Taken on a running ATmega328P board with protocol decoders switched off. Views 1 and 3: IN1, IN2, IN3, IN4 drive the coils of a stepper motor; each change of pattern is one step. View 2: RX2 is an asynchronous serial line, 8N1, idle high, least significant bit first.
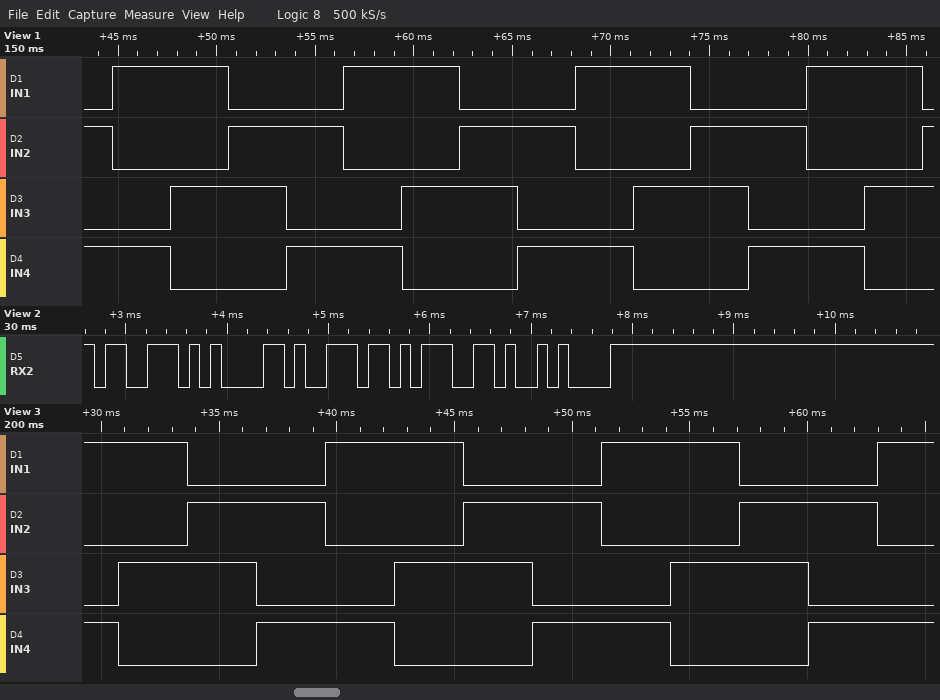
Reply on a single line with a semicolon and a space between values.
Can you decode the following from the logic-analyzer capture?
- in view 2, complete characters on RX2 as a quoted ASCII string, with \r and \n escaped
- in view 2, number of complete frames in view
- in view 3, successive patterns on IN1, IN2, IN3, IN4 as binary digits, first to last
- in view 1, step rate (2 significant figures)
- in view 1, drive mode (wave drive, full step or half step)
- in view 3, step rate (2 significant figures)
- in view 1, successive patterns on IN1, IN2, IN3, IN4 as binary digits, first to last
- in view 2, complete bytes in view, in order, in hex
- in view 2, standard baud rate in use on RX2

"sang\n"; 5; 1001 1010 0110 0101 1001 1010 0110 0101 1001 1010 0110 0101 1001; 340 steps/s; full step; 340 steps/s; 0101 1001 1010 0110 0101 1001 1010 0110 0101 1001 1010 0110 0101 1001 1010 0110; 73 61 6E 67 0A; 9600 baud
